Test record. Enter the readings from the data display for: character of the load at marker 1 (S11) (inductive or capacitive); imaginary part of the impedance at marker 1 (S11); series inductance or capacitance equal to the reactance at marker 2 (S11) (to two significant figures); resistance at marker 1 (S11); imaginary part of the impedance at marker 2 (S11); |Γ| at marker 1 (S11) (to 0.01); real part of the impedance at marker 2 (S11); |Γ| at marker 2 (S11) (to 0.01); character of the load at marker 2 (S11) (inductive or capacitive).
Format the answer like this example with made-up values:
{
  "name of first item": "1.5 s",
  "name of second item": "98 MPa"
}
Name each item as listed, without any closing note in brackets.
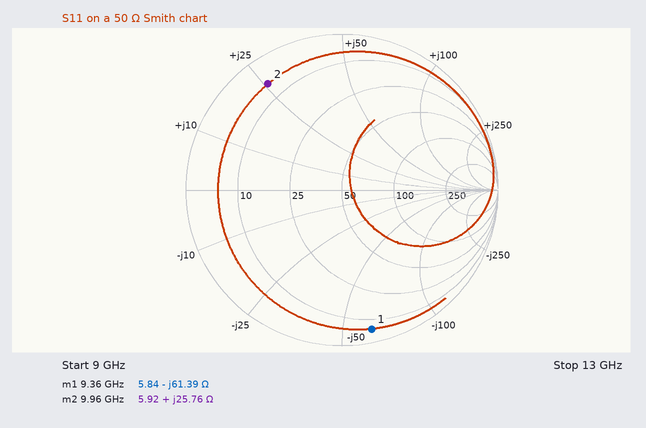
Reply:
{
  "character of the load at marker 1 (S11)": "capacitive",
  "imaginary part of the impedance at marker 1": "-61.39 Ω",
  "series inductance or capacitance equal to the reactance at marker 2 (S11)": "410 pH",
  "resistance at marker 1": "5.84 Ω",
  "imaginary part of the impedance at marker 2": "+25.76 Ω",
  "|Γ| at marker 1 (S11)": "0.91",
  "real part of the impedance at marker 2": "5.92 Ω",
  "|Γ| at marker 2 (S11)": "0.83",
  "character of the load at marker 2 (S11)": "inductive"
}
